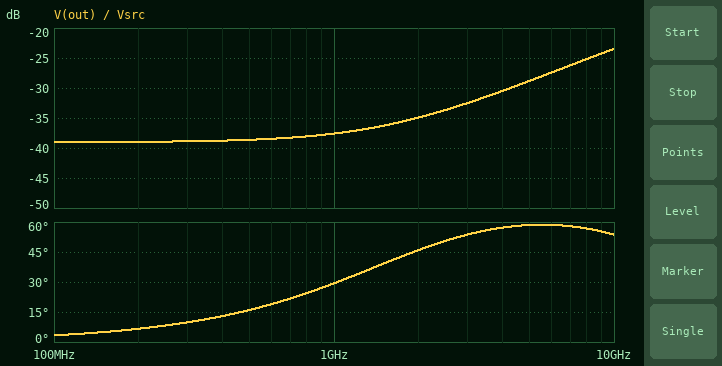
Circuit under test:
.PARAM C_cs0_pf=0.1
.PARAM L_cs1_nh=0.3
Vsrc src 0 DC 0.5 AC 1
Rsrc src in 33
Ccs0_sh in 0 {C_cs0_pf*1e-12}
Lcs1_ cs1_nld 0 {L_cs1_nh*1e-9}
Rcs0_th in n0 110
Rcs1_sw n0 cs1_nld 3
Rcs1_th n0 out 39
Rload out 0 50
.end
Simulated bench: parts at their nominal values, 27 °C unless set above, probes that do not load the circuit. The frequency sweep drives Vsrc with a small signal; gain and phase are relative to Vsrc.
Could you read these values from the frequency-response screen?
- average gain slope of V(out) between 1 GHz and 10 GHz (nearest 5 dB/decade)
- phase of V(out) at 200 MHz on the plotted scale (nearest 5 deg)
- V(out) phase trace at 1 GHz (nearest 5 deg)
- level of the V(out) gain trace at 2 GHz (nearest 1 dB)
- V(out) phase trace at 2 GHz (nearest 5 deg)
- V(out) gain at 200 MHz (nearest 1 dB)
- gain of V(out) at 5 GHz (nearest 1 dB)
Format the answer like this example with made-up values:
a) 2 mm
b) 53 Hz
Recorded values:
a) 15 dB/decade
b) 5 deg
c) 30 deg
d) -35 dB
e) 45 deg
f) -39 dB
g) -29 dB
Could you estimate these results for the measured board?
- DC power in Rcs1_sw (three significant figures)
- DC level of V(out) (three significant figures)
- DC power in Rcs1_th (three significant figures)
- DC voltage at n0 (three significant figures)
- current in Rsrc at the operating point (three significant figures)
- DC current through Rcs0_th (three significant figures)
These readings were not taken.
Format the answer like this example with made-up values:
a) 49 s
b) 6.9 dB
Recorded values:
a) 33.0 µW
b) 5.59 mV
c) 487 nW
d) 9.95 mV
e) 3.43 mA
f) 3.43 mA
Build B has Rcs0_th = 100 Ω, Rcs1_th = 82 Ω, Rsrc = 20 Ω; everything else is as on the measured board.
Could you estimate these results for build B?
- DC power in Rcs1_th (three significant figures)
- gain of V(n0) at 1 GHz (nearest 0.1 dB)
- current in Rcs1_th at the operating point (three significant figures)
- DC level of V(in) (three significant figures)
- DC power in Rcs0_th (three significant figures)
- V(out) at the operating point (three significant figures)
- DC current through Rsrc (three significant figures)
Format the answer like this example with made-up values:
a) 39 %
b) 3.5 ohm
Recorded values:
a) 670 nW
b) -31.0 dB
c) 90.4 µA
d) 419 mV
e) 1.65 mW
f) 4.52 mV
g) 4.07 mA
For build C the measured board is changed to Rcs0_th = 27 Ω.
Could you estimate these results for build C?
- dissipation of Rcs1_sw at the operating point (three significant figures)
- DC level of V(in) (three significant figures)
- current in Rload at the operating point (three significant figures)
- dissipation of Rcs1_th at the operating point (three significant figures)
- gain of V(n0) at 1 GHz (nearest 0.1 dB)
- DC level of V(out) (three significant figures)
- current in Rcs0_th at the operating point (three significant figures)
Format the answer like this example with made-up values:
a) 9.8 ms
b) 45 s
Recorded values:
a) 177 µW
b) 238 mV
c) 259 µA
d) 2.62 µW
e) -25.3 dB
f) 13.0 mV
g) 7.95 mA
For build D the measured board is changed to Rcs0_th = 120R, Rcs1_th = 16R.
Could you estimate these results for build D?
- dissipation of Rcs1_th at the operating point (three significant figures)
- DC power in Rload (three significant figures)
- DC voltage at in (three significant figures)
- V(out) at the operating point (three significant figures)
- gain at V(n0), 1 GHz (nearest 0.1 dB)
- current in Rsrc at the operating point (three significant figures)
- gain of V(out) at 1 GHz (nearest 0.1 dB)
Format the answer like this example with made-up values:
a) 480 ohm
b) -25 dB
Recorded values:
a) 311 nW
b) 973 nW
c) 394 mV
d) 6.97 mV
e) -33.3 dB
f) 3.21 mA
g) -35.7 dB
